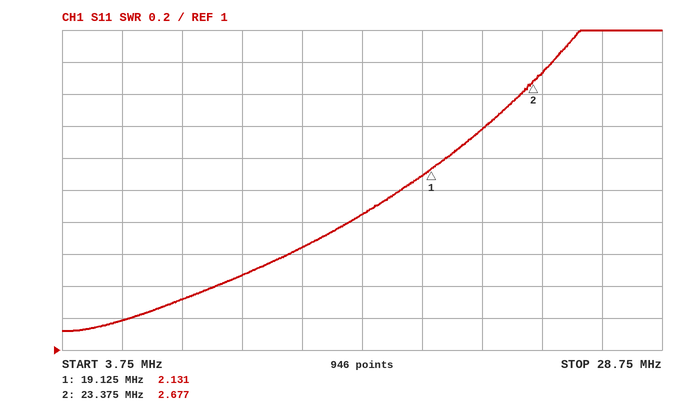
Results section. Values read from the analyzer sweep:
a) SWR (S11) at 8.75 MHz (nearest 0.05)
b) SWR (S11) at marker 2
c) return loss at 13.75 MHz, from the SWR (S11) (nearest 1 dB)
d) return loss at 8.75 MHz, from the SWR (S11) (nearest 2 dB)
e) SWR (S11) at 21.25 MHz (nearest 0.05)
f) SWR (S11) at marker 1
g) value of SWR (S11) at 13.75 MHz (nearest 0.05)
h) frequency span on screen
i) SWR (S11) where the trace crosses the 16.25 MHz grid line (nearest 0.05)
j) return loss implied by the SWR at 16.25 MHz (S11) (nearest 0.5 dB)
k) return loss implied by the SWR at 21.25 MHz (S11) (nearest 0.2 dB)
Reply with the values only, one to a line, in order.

1.30
2.677
12 dB
18 dB
2.40
2.131
1.65
25 MHz
1.85
10.5 dB
7.8 dB
